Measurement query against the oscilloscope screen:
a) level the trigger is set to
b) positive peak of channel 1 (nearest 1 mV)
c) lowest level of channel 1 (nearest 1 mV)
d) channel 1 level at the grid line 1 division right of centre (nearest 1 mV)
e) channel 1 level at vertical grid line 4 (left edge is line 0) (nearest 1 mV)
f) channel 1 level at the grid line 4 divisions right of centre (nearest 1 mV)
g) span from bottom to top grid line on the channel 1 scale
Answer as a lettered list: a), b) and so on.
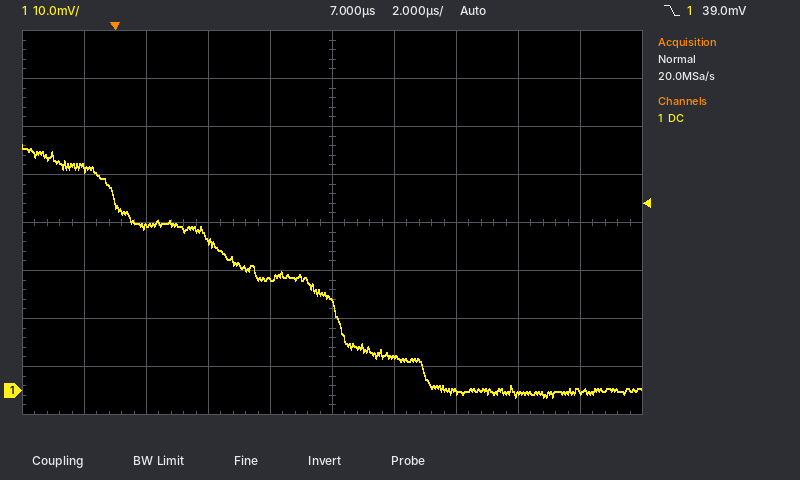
a) 39.0 mV
b) 51 mV
c) -1 mV
d) 7 mV
e) 23 mV
f) 0 mV
g) 80 mV
